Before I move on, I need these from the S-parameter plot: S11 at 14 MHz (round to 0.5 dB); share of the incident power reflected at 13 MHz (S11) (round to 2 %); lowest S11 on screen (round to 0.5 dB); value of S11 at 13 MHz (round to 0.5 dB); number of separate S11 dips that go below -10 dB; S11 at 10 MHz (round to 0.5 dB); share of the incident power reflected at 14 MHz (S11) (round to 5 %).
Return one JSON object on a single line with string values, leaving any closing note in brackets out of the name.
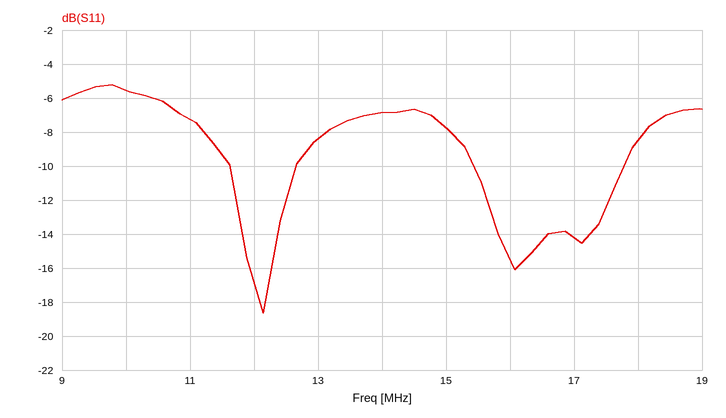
{"S11 at 14 MHz": "-7.0 dB", "share of the incident power reflected at 13 MHz (S11)": "14 %", "lowest S11 on screen": "-18.5 dB", "value of S11 at 13 MHz": "-8.5 dB", "number of separate S11 dips that go below -10 dB": "2", "S11 at 10 MHz": "-5.5 dB", "share of the incident power reflected at 14 MHz (S11)": "20 %"}
